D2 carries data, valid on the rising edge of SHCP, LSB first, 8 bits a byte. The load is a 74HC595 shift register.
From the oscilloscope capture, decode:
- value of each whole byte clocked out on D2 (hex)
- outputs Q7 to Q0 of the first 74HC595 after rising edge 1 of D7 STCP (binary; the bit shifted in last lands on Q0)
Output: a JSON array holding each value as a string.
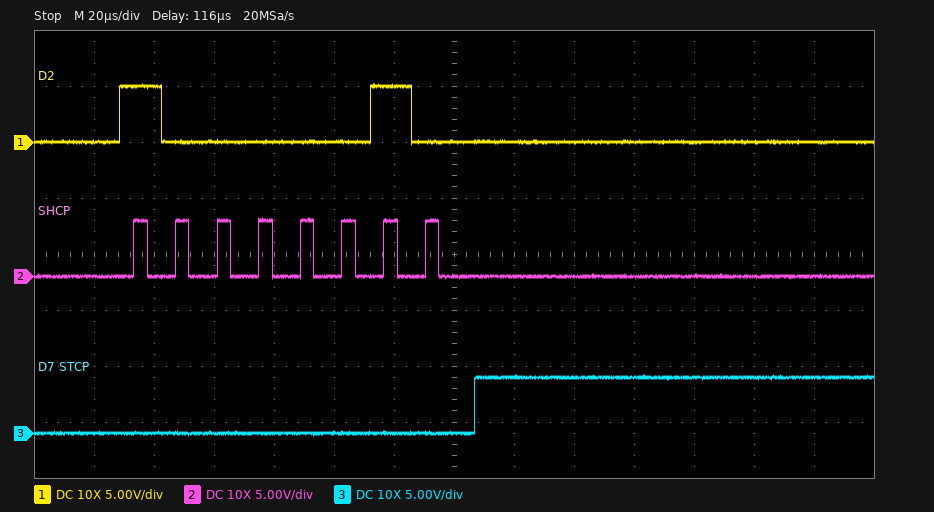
["41", "10000010"]
